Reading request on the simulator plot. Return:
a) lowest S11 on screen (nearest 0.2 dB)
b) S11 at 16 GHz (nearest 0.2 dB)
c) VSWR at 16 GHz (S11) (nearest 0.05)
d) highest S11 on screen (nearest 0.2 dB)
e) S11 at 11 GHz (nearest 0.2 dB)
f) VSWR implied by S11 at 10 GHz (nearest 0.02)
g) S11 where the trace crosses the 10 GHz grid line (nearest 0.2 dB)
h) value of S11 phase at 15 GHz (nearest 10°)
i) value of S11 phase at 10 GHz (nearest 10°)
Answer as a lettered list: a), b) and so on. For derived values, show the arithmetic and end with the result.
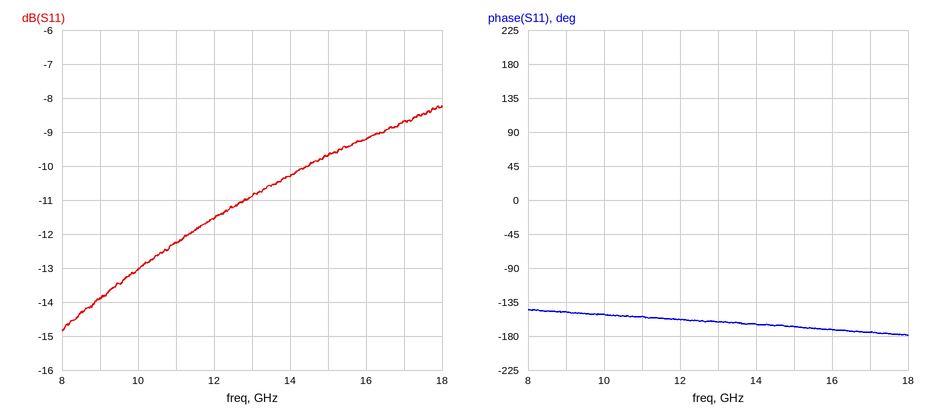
a) -14.8 dB
b) -9.2 dB
c) |Γ| = 10^(-9.2/20) = 0.3467; VSWR = (1 + 0.3467)/(1 − 0.3467) ≈ 2.06, so 2.05 to the nearest 0.05
d) -8.2 dB
e) -12.2 dB
f) |Γ| = 10^(-13/20) = 0.2239; VSWR = (1 + 0.2239)/(1 − 0.2239) ≈ 1.58
g) -13.0 dB
h) -170°
i) -150°
